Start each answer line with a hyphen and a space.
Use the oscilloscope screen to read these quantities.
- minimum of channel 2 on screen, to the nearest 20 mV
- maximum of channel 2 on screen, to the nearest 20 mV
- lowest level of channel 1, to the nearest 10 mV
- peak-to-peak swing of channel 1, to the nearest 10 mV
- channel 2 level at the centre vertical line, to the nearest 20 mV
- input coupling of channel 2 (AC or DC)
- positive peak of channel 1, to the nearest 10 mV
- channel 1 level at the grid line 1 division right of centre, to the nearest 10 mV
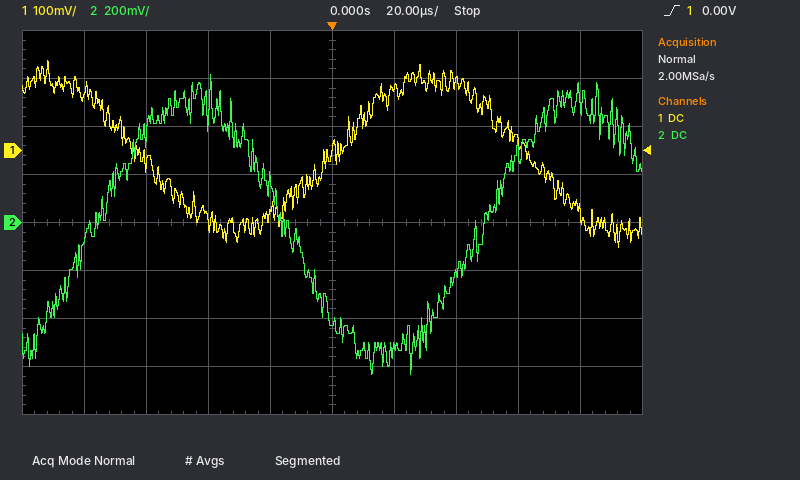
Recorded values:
- -640 mV
- 620 mV
- -200 mV
- 390 mV
- -420 mV
- DC
- 190 mV
- 130 mV
